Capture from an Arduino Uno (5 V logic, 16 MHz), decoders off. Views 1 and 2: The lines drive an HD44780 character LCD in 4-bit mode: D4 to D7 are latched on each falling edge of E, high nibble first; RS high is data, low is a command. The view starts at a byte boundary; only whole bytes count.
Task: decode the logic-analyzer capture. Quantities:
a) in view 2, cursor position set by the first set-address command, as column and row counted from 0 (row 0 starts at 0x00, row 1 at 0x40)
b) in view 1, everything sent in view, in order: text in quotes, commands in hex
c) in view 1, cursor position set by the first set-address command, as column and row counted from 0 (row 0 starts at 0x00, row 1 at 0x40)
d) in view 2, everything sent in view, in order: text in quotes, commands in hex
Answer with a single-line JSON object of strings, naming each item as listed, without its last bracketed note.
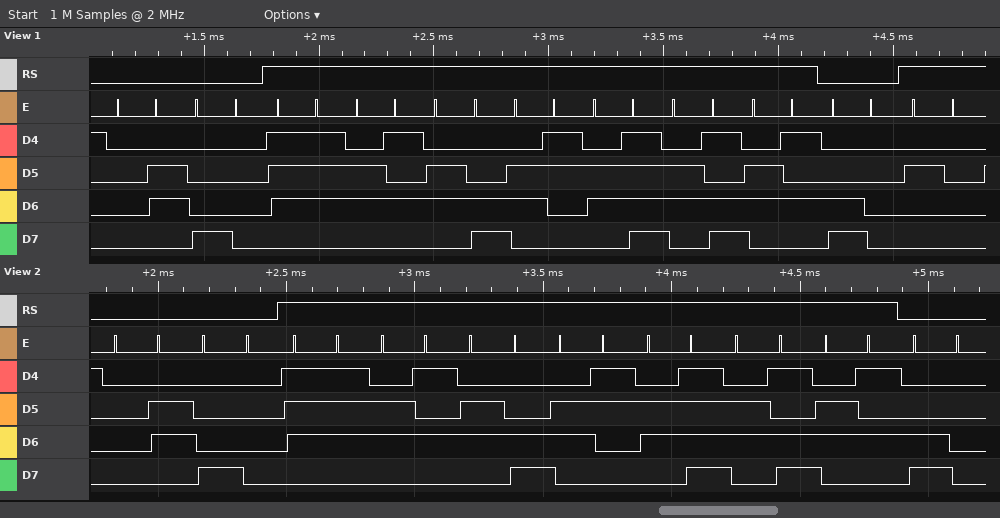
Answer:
{"in view 2, cursor position set by the first set-address command, as column and row counted from 0": "column 0, row 0", "in view 1, everything sent in view, in order: text in quotes, commands in hex": "0x06 0x80 \"welcome\" 0xC0 \" \"", "in view 1, cursor position set by the first set-address command, as column and row counted from 0": "column 0, row 0", "in view 2, everything sent in view, in order: text in quotes, commands in hex": "0x06 0x80 \"welcome\" 0xC0"}
